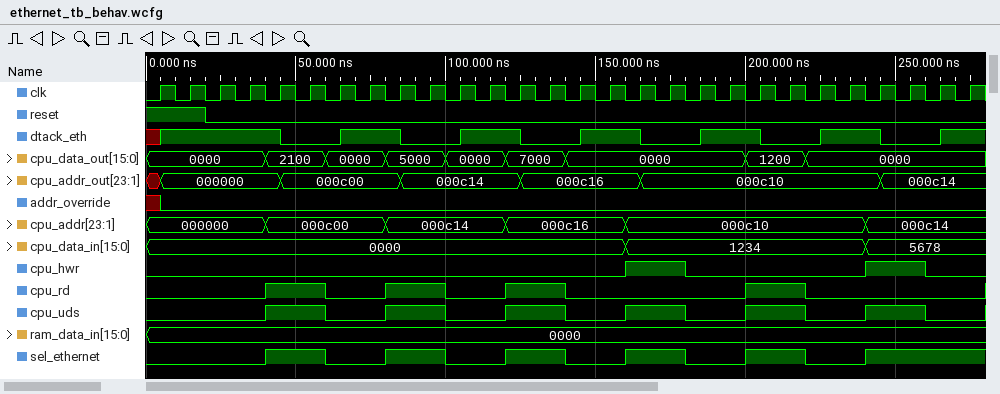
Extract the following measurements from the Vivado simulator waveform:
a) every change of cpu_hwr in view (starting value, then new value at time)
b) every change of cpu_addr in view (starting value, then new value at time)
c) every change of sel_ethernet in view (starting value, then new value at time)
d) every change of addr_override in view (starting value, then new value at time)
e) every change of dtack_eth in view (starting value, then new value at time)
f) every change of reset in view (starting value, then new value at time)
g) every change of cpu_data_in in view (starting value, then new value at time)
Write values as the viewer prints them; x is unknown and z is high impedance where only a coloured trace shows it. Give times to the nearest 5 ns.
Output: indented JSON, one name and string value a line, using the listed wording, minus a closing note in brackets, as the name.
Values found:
{
  "every change of cpu_hwr in view": "0, 1 at 160 ns, 0 at 180 ns, 1 at 240 ns, 0 at 260 ns",
  "every change of cpu_addr in view": "000000, 000c00 at 40 ns, 000c14 at 80 ns, 000c16 at 120 ns, 000c10 at 160 ns, 000c14 at 240 ns",
  "every change of sel_ethernet in view": "0, 1 at 40 ns, 0 at 60 ns, 1 at 80 ns, 0 at 100 ns, 1 at 120 ns, 0 at 140 ns, 1 at 160 ns, 0 at 180 ns, 1 at 200 ns, 0 at 220 ns, 1 at 240 ns",
  "every change of addr_override in view": "x, 0 at 5 ns",
  "every change of dtack_eth in view": "x, 1 at 5 ns, 0 at 45 ns, 1 at 65 ns, 0 at 85 ns, 1 at 105 ns, 0 at 125 ns, 1 at 145 ns, 0 at 165 ns, 1 at 185 ns, 0 at 205 ns, 1 at 225 ns, 0 at 245 ns, 1 at 265 ns",
  "every change of reset in view": "1, 0 at 20 ns",
  "every change of cpu_data_in in view": "0000, 1234 at 160 ns, 5678 at 240 ns"
}
